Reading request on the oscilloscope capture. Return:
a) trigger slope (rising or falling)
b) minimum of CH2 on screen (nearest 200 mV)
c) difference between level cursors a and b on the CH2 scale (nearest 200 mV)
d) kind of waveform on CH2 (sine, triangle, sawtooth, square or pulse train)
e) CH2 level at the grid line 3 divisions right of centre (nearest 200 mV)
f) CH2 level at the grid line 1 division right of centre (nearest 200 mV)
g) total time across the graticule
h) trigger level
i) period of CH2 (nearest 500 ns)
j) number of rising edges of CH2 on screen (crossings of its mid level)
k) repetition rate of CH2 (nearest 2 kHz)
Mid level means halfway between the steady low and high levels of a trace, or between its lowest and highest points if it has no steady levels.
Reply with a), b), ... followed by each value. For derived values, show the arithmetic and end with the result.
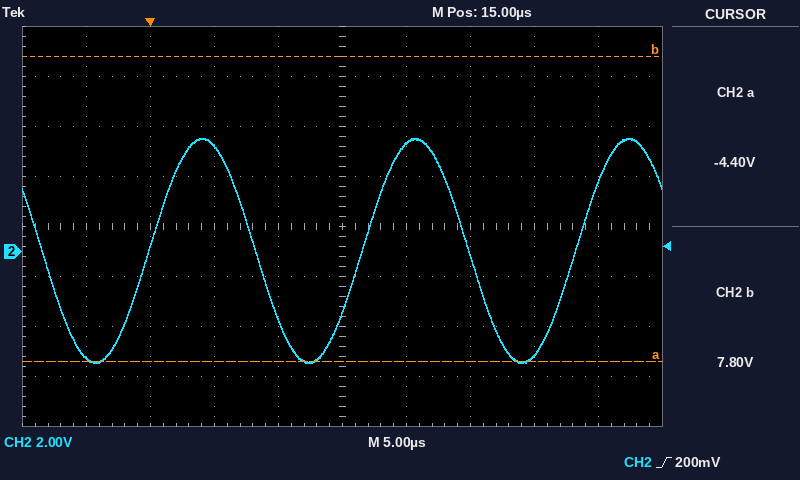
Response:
a) rising
b) -4.4 V
c) 12.2 V
d) sine
e) -4.2 V
f) 4.4 V
g) 50 µs
h) 200 mV
i) 16.5 µs
j) 3
k) 1 / 16.5 µs ≈ 60.6 kHz, so 60 kHz to the nearest 2 kHz
